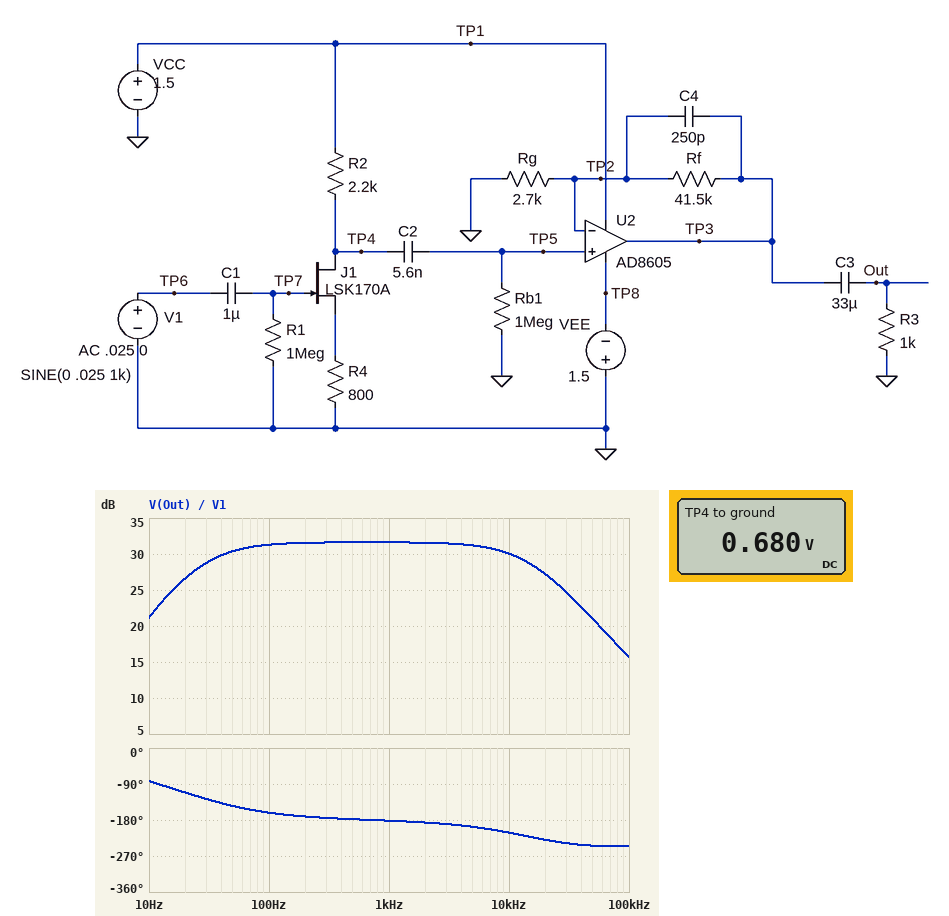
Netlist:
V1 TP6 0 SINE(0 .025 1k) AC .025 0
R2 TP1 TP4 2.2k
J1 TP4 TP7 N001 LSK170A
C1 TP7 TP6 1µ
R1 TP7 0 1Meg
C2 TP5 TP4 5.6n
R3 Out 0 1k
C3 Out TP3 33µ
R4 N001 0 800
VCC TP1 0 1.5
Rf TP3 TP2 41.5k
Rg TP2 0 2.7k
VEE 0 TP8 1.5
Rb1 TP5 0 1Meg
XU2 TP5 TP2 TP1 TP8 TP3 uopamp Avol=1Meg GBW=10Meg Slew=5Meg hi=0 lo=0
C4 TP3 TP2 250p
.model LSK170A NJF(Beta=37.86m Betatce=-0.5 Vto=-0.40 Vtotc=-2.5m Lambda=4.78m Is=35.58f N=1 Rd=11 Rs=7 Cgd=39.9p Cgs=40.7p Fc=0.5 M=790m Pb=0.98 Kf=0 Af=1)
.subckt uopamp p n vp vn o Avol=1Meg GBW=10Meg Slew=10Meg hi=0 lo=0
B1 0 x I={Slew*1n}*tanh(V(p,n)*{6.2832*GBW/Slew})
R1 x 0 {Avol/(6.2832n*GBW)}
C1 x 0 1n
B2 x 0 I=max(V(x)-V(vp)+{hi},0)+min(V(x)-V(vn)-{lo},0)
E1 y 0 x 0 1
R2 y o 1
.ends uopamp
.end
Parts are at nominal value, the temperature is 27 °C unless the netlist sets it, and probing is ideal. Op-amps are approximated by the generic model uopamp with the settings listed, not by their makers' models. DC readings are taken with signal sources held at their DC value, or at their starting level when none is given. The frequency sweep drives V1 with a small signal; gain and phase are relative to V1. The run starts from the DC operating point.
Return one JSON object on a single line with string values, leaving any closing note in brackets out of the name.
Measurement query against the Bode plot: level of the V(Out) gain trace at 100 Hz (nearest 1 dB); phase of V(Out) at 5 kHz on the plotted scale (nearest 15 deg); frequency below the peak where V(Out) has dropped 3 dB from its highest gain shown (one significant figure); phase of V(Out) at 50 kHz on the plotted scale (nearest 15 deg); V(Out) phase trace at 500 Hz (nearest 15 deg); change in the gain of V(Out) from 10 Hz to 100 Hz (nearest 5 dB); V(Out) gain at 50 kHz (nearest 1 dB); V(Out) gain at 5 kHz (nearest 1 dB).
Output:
{"level of the V(Out) gain trace at 100 Hz": "31 dB", "phase of V(Out) at 5 kHz on the plotted scale": "-195 deg", "frequency below the peak where V(Out) has dropped 3 dB from its highest gain shown": "30 Hz", "phase of V(Out) at 50 kHz on the plotted scale": "-240 deg", "V(Out) phase trace at 500 Hz": "-180 deg", "change in the gain of V(Out) from 10 Hz to 100 Hz": "10 dB", "V(Out) gain at 50 kHz": "21 dB", "V(Out) gain at 5 kHz": "31 dB"}
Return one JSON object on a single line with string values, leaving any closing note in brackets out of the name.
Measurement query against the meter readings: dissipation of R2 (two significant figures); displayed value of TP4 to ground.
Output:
{"dissipation of R2": "310 µW", "displayed value of TP4 to ground": "0.680 V"}
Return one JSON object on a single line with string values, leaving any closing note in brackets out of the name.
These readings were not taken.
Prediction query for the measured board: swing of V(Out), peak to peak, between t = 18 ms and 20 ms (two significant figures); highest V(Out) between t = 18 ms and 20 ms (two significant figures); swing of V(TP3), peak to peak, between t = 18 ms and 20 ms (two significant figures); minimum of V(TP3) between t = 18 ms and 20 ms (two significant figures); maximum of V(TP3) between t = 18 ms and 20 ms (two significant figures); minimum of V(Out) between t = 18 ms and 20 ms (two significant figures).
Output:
{"swing of V(Out), peak to peak, between t = 18 ms and 20 ms": "1.9 V", "highest V(Out) between t = 18 ms and 20 ms": "950 mV", "swing of V(TP3), peak to peak, between t = 18 ms and 20 ms": "1.9 V", "minimum of V(TP3) between t = 18 ms and 20 ms": "-950 mV", "maximum of V(TP3) between t = 18 ms and 20 ms": "950 mV", "minimum of V(Out) between t = 18 ms and 20 ms": "-950 mV"}
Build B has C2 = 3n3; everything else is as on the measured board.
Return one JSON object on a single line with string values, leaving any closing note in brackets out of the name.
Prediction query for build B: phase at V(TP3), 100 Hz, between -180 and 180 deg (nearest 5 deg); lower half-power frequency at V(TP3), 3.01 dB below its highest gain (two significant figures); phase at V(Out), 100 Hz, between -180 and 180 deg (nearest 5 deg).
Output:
{"phase at V(TP3), 100 Hz, between -180 and 180 deg": "-155 deg", "lower half-power frequency at V(TP3), 3.01 dB below its highest gain": "48 Hz", "phase at V(Out), 100 Hz, between -180 and 180 deg": "-150 deg"}
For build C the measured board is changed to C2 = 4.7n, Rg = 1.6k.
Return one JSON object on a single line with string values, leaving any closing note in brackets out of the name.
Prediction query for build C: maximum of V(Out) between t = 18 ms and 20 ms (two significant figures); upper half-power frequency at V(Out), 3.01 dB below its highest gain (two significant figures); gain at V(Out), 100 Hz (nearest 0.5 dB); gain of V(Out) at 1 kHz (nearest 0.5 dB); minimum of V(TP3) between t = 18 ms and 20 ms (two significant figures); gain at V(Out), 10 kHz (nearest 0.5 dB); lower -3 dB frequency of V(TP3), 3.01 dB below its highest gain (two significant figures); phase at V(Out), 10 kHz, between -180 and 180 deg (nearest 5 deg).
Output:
{"maximum of V(Out) between t = 18 ms and 20 ms": "1.5 V", "upper half-power frequency at V(Out), 3.01 dB below its highest gain": "15 kHz", "gain at V(Out), 100 Hz": "35.5 dB", "gain of V(Out) at 1 kHz": "36.0 dB", "minimum of V(TP3) between t = 18 ms and 20 ms": "-1.5 V", "gain at V(Out), 10 kHz": "34.5 dB", "lower -3 dB frequency of V(TP3), 3.01 dB below its highest gain": "34 Hz", "phase at V(Out), 10 kHz, between -180 and 180 deg": "145 deg"}
